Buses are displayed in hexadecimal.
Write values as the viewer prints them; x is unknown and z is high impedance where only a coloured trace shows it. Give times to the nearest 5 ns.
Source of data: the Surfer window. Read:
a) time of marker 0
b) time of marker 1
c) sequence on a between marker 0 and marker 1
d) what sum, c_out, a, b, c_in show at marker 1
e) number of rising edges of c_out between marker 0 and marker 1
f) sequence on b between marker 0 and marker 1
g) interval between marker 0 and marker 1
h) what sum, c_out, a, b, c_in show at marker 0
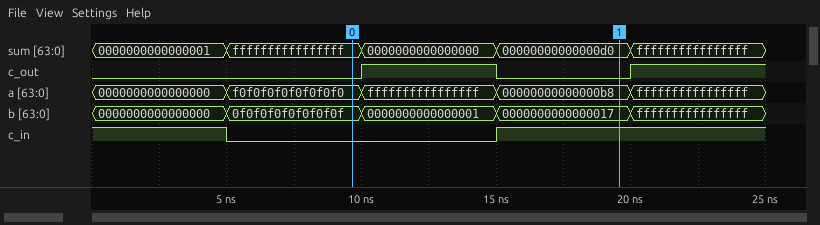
10 ns
20 ns
f0f0f0f0f0f0f0f0, ffffffffffffffff, 00000000000000b8
sum=00000000000000d0, c_out=0, a=00000000000000b8, b=0000000000000017, c_in=1
1
0f0f0f0f0f0f0f0f, 0000000000000001, 0000000000000017
10 ns
sum=ffffffffffffffff, c_out=0, a=f0f0f0f0f0f0f0f0, b=0f0f0f0f0f0f0f0f, c_in=0
